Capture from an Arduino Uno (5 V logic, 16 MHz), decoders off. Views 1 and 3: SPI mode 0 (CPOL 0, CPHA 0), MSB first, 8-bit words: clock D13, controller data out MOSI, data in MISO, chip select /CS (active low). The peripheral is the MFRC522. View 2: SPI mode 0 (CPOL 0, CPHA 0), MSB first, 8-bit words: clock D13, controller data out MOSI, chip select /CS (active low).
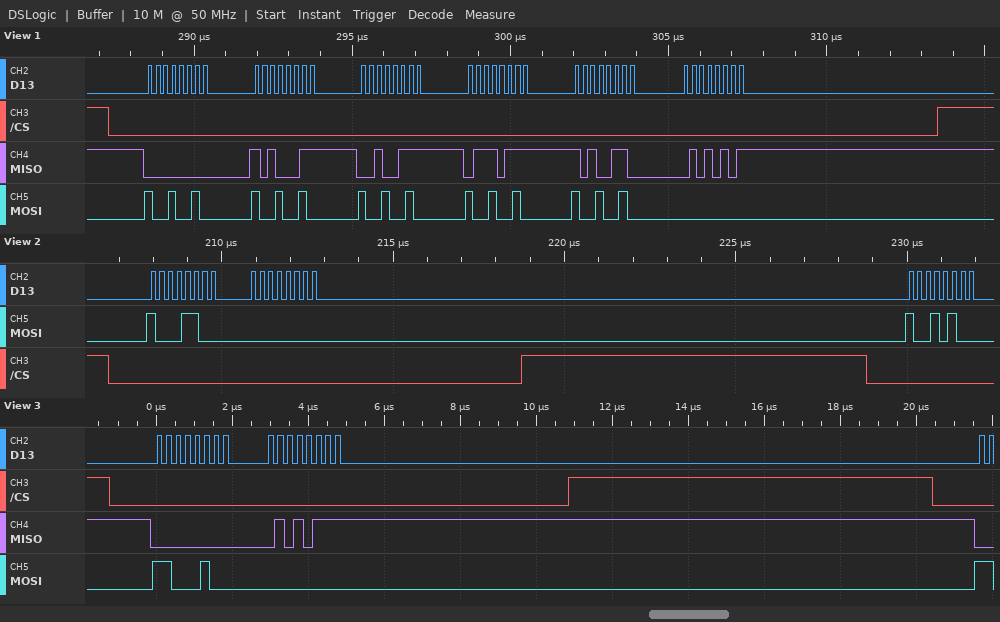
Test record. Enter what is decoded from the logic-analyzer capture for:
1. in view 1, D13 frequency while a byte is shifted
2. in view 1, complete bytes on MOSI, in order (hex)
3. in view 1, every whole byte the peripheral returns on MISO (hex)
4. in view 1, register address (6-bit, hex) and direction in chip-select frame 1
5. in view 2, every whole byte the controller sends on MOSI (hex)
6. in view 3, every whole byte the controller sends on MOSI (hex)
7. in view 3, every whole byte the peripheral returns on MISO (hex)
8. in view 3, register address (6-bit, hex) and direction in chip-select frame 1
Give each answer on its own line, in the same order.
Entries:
4 MHz
92 92 92 92 92 00
00 A3 27 77 A6 55
0x09 read
0x8C 0x00 0x94
C4 00
00 57
0x22 read
